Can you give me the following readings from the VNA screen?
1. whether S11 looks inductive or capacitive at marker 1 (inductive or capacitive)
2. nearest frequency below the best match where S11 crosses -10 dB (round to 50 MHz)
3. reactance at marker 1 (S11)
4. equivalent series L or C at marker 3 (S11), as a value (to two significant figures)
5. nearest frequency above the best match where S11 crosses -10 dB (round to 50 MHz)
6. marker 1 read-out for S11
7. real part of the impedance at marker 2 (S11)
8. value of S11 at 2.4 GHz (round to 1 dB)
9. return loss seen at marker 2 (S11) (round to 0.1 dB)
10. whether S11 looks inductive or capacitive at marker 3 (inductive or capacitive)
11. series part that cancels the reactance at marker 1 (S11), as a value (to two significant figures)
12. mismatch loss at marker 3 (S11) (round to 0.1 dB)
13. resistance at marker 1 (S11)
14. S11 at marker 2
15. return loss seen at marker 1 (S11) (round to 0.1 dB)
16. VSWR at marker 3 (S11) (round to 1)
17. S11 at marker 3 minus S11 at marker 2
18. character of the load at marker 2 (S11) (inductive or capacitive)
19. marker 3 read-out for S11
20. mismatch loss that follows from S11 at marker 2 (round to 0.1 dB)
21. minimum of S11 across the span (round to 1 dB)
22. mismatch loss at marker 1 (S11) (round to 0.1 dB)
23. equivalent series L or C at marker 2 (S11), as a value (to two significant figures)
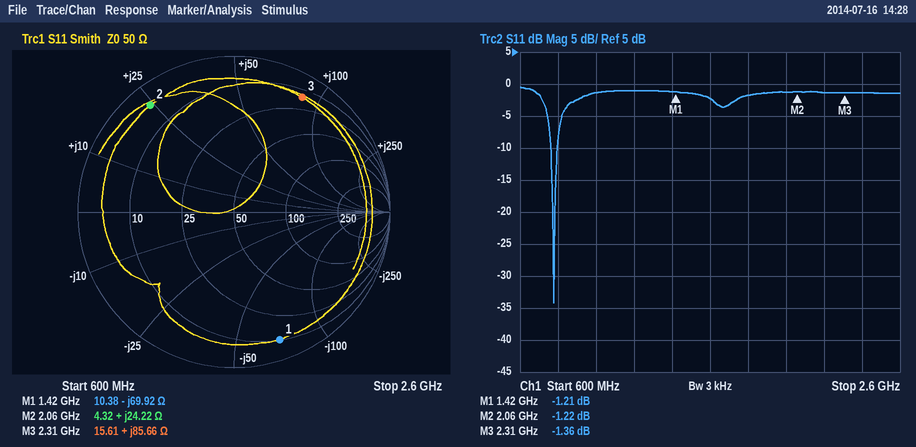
capacitive
750 MHz
-69.92 Ω
5.9 nH
800 MHz
-1.21 dB
4.32 Ω
-1 dB
1.2 dB
inductive
7.8 nH
5.7 dB
10.38 Ω
-1.22 dB
1.2 dB
13
-0.14 dB
inductive
-1.36 dB
6.1 dB
-34 dB
6.1 dB
1.9 nH
